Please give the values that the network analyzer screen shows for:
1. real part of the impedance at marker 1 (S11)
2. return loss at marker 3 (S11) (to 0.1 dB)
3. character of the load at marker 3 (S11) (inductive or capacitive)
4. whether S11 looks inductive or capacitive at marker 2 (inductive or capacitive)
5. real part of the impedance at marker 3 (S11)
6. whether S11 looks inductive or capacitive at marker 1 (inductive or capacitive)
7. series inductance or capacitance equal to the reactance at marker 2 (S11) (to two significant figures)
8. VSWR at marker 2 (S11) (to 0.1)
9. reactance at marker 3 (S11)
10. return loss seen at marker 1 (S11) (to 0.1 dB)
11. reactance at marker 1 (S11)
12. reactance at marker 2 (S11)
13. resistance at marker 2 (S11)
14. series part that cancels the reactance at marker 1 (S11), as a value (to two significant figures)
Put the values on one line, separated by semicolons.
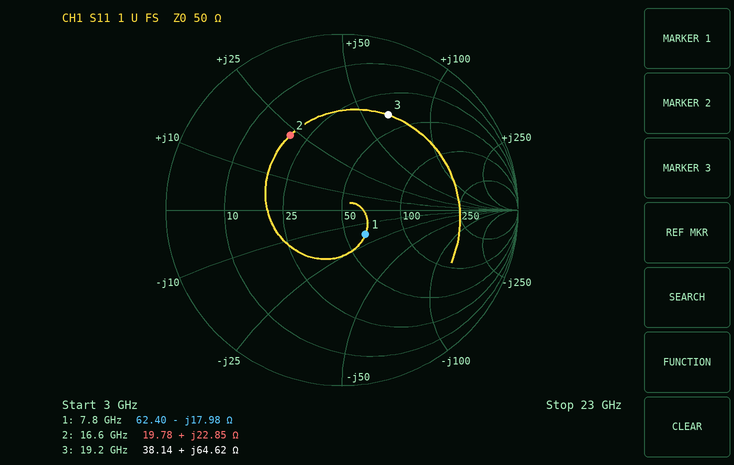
62.40 Ω; 4.4 dB; inductive; inductive; 38.14 Ω; capacitive; 220 pH; 3.1; +64.62 Ω; 14.3 dB; -17.98 Ω; +22.85 Ω; 19.78 Ω; 370 pH
